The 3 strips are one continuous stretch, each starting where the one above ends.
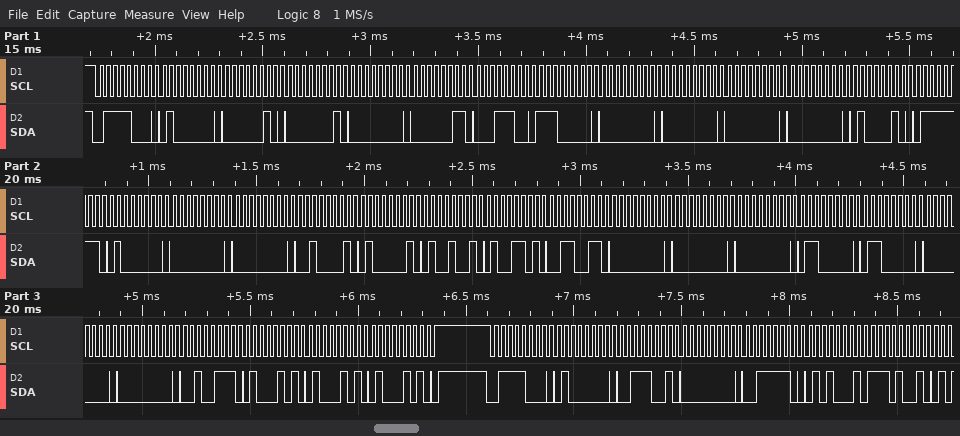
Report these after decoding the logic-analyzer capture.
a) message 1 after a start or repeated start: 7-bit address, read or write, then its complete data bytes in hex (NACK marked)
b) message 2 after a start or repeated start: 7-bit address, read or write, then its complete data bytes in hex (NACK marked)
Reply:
0x3C write: 40 02 01 00 03 1C E0 00 00 00 00 42 7F 40 00 00 21 41 49 4D 33 00 00 00 60 60 00 00 27 45 45 45
0x3C write: 40 39 00 3E 51 E9
